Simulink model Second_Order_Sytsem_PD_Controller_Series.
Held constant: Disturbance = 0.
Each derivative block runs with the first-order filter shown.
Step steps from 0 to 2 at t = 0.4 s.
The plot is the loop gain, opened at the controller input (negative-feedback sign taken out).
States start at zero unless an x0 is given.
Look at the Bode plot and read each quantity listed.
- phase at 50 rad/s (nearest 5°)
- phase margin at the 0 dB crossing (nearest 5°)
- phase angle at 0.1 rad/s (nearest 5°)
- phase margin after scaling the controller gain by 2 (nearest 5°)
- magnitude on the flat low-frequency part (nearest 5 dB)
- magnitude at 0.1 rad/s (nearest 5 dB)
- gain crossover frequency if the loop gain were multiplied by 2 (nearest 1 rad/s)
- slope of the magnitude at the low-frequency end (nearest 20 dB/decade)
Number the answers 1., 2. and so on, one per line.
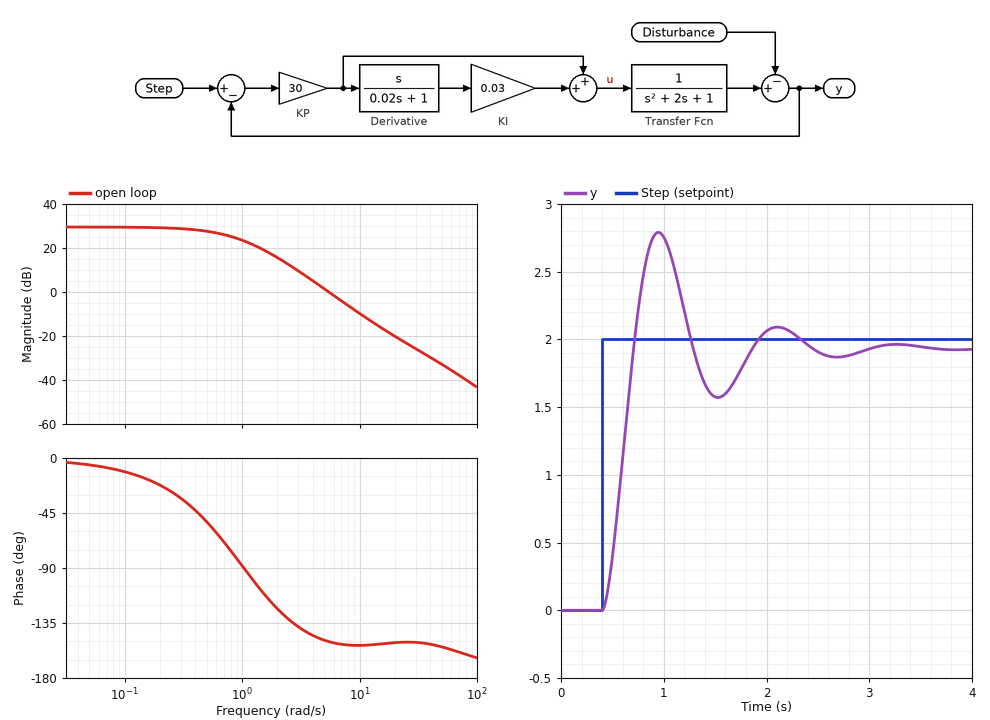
1. -155°
2. 30°
3. -10°
4. 25°
5. 30 dB
6. 30 dB
7. 8 rad/s
8. 0 dB/decade
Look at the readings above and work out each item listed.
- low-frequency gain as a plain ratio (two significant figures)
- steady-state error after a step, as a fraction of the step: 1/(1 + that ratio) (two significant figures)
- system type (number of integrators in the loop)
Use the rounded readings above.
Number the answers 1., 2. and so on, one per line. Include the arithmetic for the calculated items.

1. 10^(30 / 20) = 32
2. 1 / (1 + 32) = 0.030
3. 0
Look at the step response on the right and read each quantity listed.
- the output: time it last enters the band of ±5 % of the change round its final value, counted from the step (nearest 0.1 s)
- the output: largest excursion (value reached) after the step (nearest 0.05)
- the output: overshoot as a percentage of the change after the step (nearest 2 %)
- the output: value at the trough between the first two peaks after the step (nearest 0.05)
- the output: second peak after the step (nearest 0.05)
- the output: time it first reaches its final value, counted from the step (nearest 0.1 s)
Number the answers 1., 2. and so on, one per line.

1. 1.9 s
2. 2.80
3. 44 %
4. 1.55
5. 2.10
6. 0.3 s
